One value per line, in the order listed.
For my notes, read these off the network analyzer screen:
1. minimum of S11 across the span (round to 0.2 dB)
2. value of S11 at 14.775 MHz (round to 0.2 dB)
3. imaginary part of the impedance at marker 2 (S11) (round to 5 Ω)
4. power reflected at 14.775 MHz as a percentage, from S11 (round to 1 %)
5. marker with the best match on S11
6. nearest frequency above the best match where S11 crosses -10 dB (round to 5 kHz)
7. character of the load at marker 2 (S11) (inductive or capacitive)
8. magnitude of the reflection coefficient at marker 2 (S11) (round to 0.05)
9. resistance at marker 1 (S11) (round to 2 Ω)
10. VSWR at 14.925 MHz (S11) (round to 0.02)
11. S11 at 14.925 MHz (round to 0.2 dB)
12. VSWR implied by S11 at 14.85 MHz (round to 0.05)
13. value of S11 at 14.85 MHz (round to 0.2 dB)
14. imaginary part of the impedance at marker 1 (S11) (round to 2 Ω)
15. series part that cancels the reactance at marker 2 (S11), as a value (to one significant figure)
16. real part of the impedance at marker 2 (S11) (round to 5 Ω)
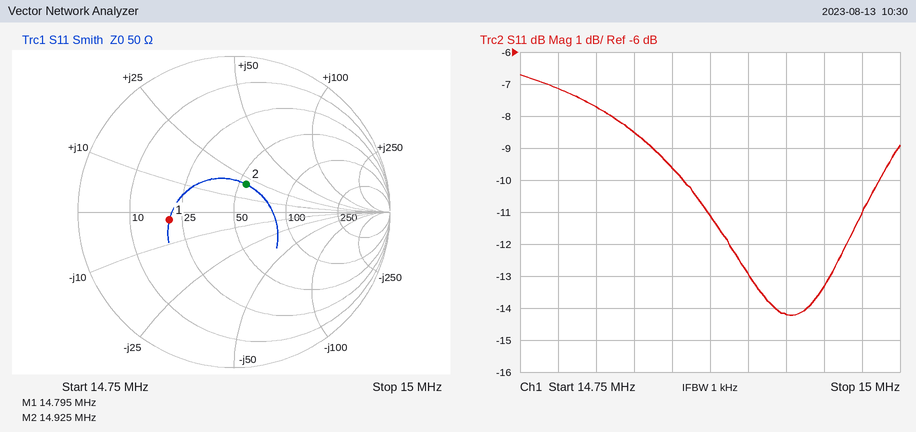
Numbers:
-14.2 dB
-7.2 dB
+20 Ω
19 %
marker 2
14.985 MHz
inductive
0.20
20 Ω
1.48
-14.2 dB
2.00
-9.6 dB
-2 Ω
500 pF
55 Ω
